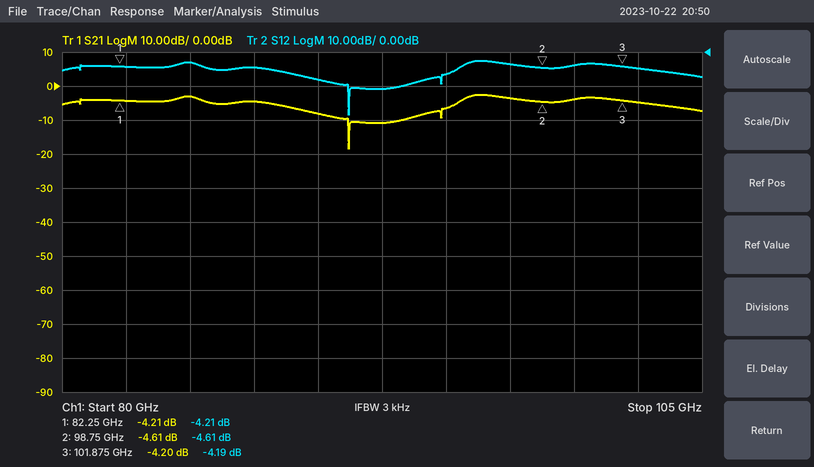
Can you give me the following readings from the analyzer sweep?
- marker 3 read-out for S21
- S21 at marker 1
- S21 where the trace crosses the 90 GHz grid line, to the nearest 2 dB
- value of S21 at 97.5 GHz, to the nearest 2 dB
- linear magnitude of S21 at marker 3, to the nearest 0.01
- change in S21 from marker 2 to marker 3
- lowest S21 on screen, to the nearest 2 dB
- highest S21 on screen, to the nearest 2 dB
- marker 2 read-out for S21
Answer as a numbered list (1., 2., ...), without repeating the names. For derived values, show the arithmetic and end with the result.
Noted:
1. -4.20 dB
2. -4.21 dB
3. -8 dB
4. -4 dB
5. 10^(-4.2/20) ≈ 0.62
6. -4.2 − (-4.61) = 0.41 dB
7. -18 dB
8. -2 dB
9. -4.61 dB
